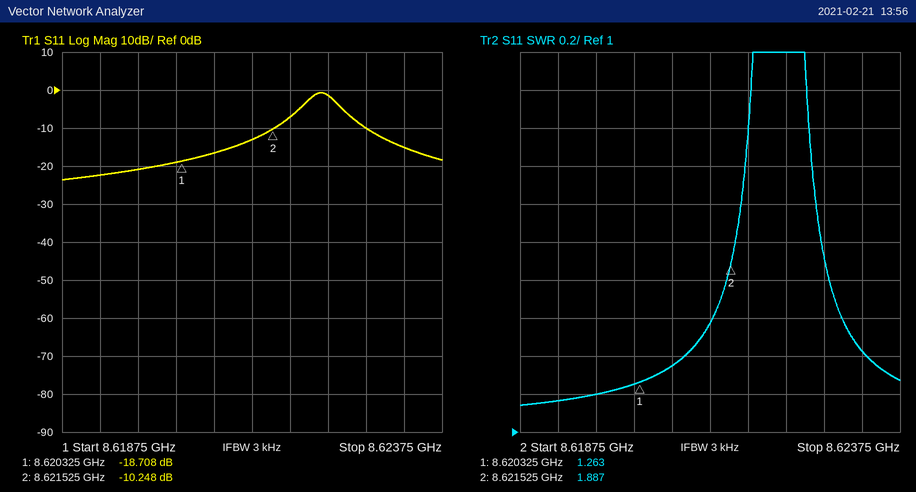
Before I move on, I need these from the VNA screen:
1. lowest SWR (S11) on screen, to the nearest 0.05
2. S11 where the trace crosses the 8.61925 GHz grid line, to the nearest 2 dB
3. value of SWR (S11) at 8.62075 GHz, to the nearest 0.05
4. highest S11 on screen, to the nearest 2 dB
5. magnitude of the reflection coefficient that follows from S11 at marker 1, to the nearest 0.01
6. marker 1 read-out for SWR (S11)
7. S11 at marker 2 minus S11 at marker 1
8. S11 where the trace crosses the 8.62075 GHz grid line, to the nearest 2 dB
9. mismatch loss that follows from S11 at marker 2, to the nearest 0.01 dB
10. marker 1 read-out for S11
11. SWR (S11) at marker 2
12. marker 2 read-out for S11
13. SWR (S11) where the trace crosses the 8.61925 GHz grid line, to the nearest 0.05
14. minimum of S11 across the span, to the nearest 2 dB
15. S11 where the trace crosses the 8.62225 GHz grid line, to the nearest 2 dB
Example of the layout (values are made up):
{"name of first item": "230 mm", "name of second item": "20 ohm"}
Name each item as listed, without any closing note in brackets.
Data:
{"lowest SWR (S11) on screen, to the nearest 0.05": "1.15", "S11 where the trace crosses the 8.61925 GHz grid line, to the nearest 2 dB": "-22 dB", "value of SWR (S11) at 8.62075 GHz, to the nearest 0.05": "1.35", "highest S11 on screen, to the nearest 2 dB": "0 dB", "magnitude of the reflection coefficient that follows from S11 at marker 1, to the nearest 0.01": "0.12", "marker 1 read-out for SWR": "1.263", "S11 at marker 2 minus S11 at marker 1": "8.460 dB", "S11 where the trace crosses the 8.62075 GHz grid line, to the nearest 2 dB": "-16 dB", "mismatch loss that follows from S11 at marker 2, to the nearest 0.01 dB": "0.43 dB", "marker 1 read-out for S11": "-18.708 dB", "SWR (S11) at marker 2": "1.887", "marker 2 read-out for S11": "-10.248 dB", "SWR (S11) where the trace crosses the 8.61925 GHz grid line, to the nearest 0.05": "1.15", "minimum of S11 across the span, to the nearest 2 dB": "-24 dB", "S11 where the trace crosses the 8.62225 GHz grid line, to the nearest 2 dB": "-2 dB"}
